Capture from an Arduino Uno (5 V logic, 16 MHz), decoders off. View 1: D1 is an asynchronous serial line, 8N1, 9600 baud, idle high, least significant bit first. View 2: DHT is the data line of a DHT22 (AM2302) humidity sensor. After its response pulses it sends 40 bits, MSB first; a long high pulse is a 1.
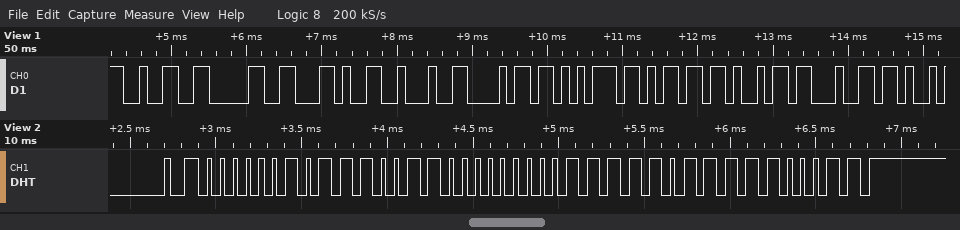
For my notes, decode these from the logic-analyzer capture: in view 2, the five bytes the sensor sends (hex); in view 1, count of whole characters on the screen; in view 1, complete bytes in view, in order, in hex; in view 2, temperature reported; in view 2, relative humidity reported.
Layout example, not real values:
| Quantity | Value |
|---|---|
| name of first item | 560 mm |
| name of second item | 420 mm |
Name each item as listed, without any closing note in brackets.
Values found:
| Quantity | Value |
|---|---|
| in view 2, the five bytes the sensor sends | 02 E6 00 FB E3 |
| in view 1, count of whole characters on the screen | 9 |
| in view 1, complete bytes in view, in order, in hex | 0x32 0x30 0x2C 0x22 0x68 0x75 0x6D 0x69 0x64 |
| in view 2, temperature reported | 25.1 °C |
| in view 2, relative humidity reported | 74.2 % |
